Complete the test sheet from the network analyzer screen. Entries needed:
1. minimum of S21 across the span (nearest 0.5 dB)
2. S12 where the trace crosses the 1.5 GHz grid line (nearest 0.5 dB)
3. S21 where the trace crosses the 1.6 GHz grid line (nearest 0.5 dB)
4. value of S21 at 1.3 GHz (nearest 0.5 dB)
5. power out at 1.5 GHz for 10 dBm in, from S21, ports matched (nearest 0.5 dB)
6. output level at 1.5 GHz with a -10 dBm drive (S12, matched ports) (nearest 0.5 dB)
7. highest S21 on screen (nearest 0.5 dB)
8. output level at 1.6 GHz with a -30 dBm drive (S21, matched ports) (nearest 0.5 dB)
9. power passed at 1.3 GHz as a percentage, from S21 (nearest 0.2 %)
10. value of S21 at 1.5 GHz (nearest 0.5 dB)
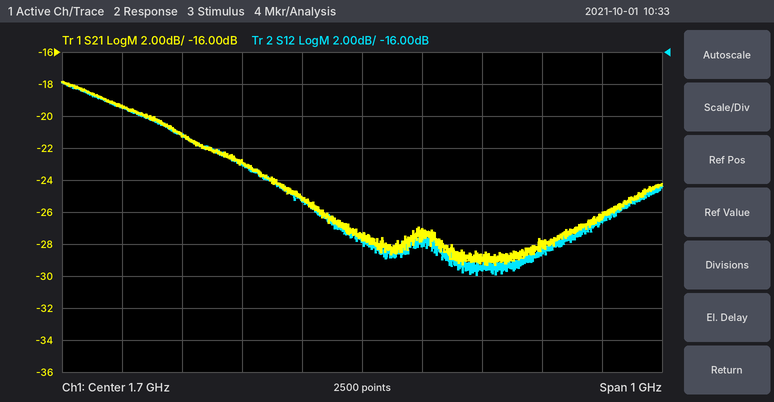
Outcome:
-29.5 dB
-23.0 dB
-25.0 dB
-19.5 dB
-13.0 dBm
-33.0 dBm
-18.0 dB
-55.0 dBm
1.2 %
-23.0 dB
